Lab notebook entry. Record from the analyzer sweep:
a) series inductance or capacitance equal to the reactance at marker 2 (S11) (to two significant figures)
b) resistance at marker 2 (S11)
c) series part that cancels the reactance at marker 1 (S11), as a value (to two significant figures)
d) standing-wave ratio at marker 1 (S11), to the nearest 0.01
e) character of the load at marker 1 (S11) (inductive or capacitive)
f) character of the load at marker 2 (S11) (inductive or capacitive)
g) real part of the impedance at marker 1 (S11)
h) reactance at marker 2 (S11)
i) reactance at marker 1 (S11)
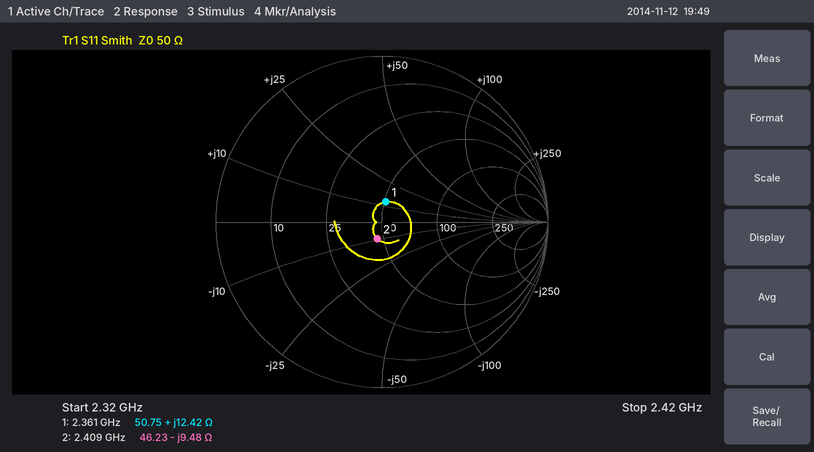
7.0 pF
46.23 Ω
5.4 pF
1.28
inductive
capacitive
50.75 Ω
-9.48 Ω
+12.42 Ω
